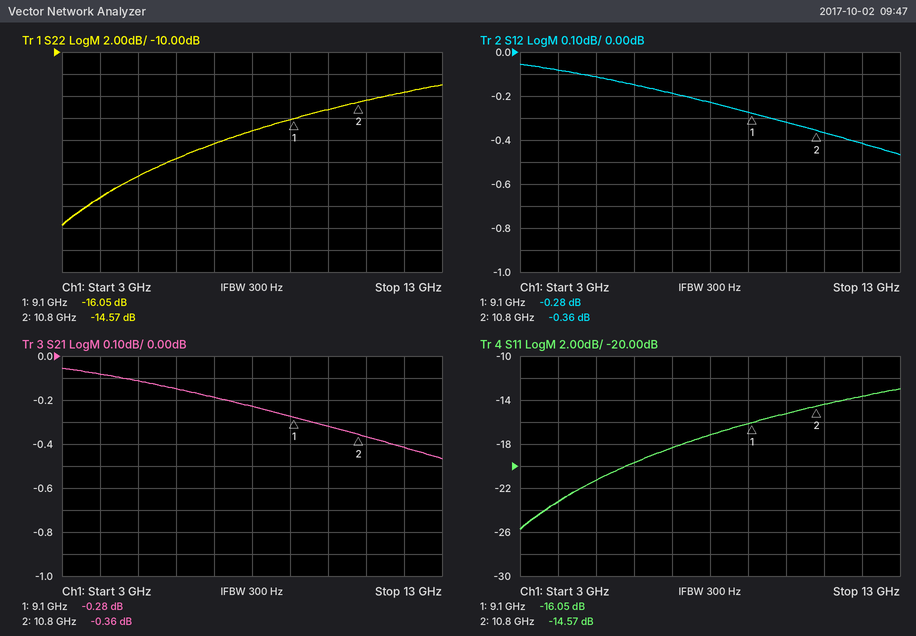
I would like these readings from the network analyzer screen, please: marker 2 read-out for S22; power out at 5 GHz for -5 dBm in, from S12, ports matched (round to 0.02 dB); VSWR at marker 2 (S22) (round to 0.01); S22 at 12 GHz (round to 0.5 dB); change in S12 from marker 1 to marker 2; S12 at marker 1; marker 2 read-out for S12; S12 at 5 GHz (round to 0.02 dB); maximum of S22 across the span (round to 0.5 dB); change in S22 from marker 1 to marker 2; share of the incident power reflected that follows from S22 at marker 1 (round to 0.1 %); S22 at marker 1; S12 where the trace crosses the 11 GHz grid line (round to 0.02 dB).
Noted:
-14.57 dB
-5.12 dBm
1.46
-13.5 dB
-0.08 dB
-0.28 dB
-0.36 dB
-0.12 dB
-13.0 dB
1.48 dB
2.5 %
-16.05 dB
-0.36 dB
